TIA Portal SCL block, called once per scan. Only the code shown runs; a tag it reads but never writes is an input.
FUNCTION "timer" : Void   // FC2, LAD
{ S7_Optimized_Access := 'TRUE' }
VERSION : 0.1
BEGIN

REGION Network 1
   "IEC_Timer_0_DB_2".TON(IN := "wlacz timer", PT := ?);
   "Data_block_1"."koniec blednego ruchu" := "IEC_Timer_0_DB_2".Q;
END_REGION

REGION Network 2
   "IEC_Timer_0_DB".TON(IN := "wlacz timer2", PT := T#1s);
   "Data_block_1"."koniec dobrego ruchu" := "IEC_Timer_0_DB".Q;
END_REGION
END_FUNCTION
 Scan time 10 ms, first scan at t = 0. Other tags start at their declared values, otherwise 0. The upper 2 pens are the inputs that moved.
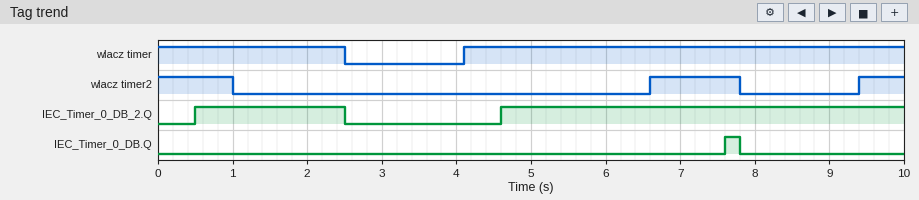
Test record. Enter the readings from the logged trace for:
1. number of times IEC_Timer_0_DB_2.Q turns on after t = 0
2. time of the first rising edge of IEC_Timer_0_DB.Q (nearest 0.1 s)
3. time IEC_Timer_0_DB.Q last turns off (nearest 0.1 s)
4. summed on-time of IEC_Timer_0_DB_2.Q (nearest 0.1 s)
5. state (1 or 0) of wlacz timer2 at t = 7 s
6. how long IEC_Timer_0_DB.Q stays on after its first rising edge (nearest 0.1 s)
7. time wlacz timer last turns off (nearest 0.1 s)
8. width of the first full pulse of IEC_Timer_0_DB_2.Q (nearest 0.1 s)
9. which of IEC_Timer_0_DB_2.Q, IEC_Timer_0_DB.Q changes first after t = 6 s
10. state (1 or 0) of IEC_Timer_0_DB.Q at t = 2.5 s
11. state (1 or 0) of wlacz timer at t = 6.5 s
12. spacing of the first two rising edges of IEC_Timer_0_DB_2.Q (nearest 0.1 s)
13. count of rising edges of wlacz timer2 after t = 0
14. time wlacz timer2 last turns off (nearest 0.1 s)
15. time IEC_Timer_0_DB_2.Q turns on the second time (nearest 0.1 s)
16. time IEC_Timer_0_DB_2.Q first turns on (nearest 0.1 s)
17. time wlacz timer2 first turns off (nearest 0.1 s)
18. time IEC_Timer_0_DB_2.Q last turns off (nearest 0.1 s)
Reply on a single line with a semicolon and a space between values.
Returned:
2; 7.6 s; 7.8 s; 7.4 s; 1; 0.2 s; 2.5 s; 2.0 s; IEC_Timer_0_DB.Q; 0; 1; 4.1 s; 2; 7.8 s; 4.6 s; 0.5 s; 1.0 s; 2.5 s
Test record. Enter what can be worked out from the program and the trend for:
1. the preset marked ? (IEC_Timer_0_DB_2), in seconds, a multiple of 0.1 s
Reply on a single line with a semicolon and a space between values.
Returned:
0.5 s
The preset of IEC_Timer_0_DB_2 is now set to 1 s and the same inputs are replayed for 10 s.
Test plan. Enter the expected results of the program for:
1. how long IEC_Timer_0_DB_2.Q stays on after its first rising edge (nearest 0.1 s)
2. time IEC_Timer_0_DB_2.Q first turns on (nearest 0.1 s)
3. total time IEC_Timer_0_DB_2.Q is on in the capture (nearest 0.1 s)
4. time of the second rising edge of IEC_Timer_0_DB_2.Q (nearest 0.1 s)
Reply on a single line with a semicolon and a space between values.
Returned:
1.5 s; 1.0 s; 6.4 s; 5.1 s
